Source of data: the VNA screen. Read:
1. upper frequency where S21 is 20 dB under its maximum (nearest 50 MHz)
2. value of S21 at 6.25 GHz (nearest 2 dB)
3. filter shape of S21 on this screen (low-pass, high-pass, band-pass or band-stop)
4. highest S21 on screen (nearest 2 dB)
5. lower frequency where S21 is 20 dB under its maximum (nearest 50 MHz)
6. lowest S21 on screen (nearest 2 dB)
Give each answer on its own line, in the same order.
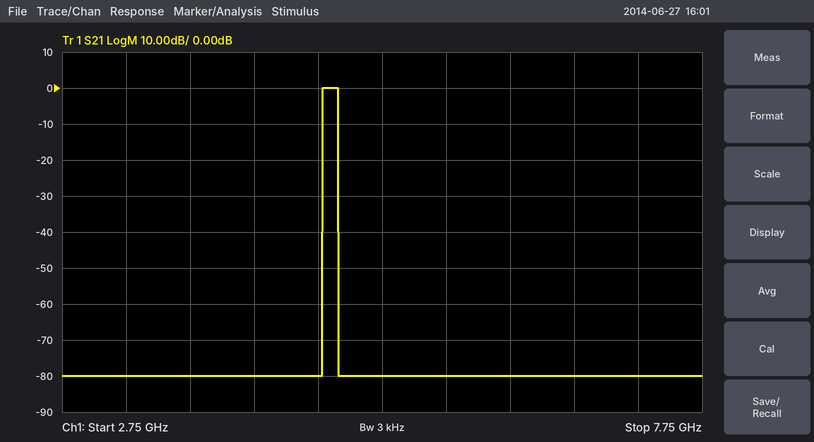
4.90 GHz
-80 dB
band-pass
0 dB
4.80 GHz
-80 dB
